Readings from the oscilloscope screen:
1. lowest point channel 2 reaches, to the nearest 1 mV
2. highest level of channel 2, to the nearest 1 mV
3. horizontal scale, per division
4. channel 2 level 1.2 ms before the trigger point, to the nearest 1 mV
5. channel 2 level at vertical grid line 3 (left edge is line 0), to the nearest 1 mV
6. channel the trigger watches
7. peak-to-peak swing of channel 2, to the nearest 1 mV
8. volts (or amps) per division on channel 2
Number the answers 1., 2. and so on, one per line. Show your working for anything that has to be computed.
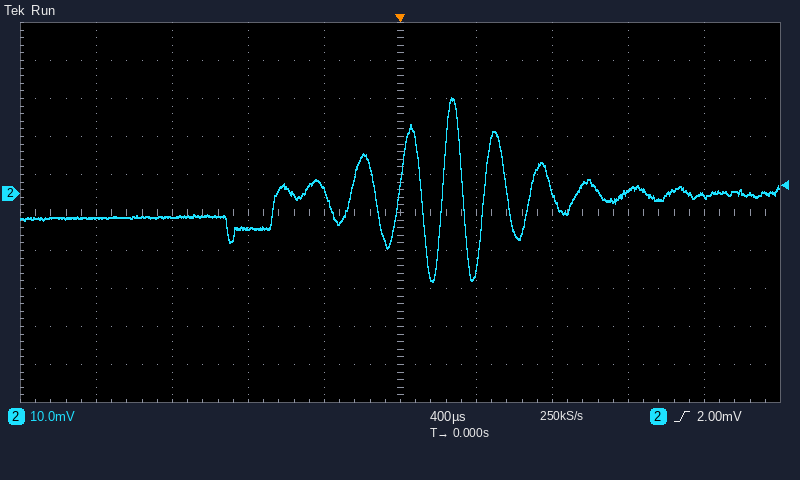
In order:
1. -23 mV
2. 25 mV
3. 400 µs
4. -6 mV
5. -9 mV
6. channel 2
7. 25 mV − (-23 mV) = 48 mV
8. 10 mV
